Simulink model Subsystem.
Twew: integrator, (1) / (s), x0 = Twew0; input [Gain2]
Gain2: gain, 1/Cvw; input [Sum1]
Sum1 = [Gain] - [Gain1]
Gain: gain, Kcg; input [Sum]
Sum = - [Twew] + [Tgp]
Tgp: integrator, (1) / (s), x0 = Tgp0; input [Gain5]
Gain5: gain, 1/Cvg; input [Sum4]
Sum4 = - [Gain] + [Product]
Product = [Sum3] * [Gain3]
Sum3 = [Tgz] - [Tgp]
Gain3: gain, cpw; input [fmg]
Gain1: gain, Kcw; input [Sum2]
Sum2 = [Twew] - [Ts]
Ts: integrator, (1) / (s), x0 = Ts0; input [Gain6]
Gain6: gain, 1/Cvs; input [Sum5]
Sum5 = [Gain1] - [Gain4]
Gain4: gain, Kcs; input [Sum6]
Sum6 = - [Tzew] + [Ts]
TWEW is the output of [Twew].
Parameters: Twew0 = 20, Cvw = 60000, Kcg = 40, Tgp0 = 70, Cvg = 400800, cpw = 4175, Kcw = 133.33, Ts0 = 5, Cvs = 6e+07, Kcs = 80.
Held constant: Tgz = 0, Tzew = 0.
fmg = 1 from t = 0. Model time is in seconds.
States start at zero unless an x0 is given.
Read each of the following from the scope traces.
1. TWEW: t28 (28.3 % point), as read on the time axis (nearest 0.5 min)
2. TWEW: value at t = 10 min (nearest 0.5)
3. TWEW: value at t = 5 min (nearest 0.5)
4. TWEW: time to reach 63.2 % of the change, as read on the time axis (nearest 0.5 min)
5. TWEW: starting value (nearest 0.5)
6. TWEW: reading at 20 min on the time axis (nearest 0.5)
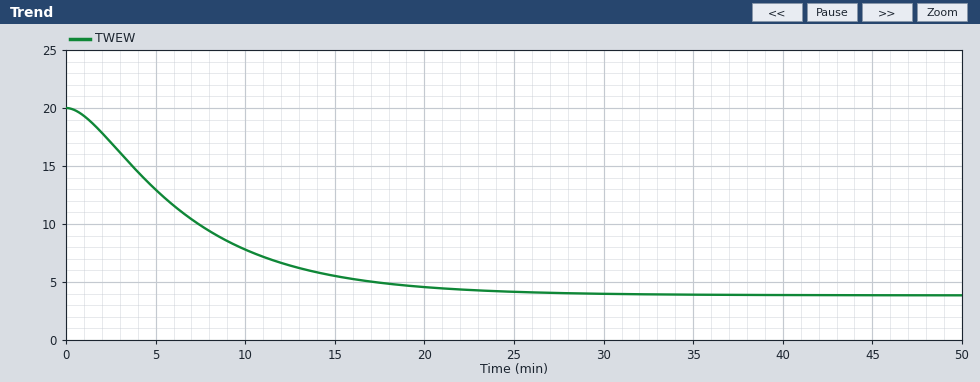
3.5 min
8.0
13.0
7.5 min
20.0
4.5
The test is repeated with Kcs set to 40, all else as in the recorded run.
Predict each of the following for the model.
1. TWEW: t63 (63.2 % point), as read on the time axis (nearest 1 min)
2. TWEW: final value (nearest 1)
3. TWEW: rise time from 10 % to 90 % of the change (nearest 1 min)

8 min
4
14 min
